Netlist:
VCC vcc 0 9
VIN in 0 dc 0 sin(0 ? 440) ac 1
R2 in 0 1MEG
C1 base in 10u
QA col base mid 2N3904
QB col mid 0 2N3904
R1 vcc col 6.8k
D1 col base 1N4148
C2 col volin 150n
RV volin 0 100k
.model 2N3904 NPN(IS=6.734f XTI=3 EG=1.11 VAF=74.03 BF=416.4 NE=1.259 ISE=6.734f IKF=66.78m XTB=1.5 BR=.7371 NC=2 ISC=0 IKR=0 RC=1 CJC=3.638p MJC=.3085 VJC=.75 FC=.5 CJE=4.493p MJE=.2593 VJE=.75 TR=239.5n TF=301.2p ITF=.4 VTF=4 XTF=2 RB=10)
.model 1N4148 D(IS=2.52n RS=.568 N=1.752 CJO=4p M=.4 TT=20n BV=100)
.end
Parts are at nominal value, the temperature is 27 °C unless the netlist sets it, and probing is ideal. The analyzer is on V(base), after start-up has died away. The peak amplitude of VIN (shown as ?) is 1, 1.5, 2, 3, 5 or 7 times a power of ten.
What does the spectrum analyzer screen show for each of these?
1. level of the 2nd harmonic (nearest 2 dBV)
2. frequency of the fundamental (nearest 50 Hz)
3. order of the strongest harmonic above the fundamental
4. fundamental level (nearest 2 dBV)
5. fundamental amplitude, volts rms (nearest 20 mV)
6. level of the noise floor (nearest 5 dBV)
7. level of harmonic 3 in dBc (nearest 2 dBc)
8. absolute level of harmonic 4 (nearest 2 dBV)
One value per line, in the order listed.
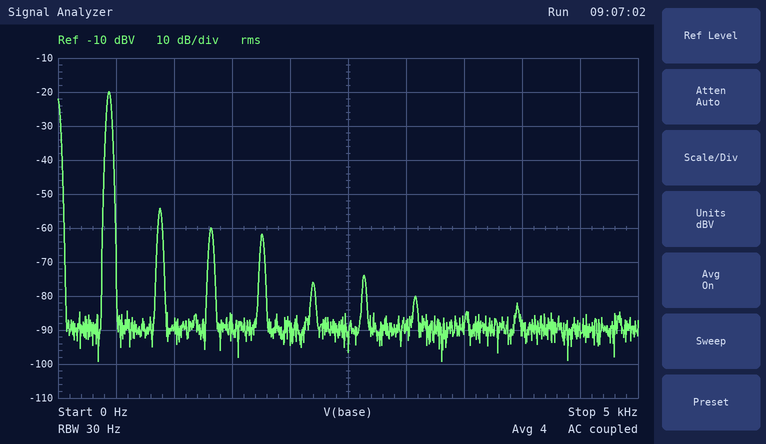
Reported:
-54 dBV
450 Hz
2
-20 dBV
100 mV
-90 dBV
-40 dBc
-62 dBV
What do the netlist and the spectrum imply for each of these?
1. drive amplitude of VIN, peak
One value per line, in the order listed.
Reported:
150 mV
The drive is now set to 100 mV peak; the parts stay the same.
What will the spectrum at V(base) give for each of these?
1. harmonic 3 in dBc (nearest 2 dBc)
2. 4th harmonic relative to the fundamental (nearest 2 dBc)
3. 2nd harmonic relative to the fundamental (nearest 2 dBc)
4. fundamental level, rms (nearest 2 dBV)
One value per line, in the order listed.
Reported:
-36 dBc
-50 dBc
-46 dBc
-24 dBV
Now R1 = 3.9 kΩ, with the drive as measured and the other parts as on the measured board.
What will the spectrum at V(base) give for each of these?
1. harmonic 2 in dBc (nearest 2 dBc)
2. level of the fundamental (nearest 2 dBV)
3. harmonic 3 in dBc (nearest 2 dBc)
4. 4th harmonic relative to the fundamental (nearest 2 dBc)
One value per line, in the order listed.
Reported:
-36 dBc
-20 dBV
-36 dBc
-40 dBc
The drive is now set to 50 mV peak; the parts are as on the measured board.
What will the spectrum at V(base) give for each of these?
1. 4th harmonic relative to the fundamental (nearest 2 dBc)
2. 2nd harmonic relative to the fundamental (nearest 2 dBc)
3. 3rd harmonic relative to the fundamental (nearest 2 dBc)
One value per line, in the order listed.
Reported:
-48 dBc
-36 dBc
-38 dBc
